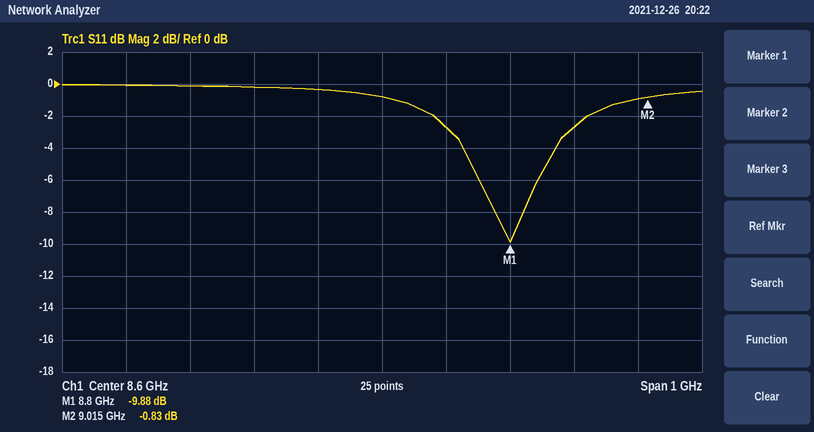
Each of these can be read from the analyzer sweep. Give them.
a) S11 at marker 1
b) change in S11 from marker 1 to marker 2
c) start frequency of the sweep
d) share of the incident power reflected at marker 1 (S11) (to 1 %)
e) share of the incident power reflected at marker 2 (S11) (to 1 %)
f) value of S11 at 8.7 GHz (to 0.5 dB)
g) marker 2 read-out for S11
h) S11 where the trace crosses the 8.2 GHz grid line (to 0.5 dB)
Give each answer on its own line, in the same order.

-9.88 dB
9.05 dB
8.1 GHz
10 %
83 %
-2.5 dB
-0.83 dB
0.0 dB
